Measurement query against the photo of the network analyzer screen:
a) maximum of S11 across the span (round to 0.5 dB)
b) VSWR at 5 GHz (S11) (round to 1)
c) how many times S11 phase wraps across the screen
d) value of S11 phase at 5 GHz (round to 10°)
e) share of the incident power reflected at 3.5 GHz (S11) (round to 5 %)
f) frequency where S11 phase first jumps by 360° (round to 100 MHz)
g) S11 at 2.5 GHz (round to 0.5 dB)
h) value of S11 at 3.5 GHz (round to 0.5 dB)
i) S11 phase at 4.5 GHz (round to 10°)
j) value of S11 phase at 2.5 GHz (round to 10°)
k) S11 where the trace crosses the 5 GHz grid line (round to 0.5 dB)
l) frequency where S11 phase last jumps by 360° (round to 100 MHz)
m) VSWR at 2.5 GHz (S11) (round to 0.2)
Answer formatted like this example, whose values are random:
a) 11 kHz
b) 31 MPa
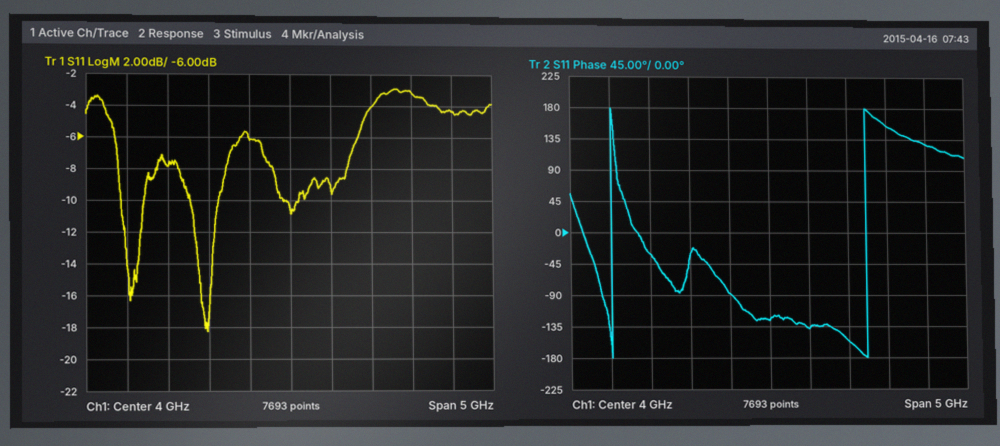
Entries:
a) -3.0 dB
b) 4
c) 2
d) -160°
e) 25 %
f) 2.0 GHz
g) -8.0 dB
h) -6.0 dB
i) -140°
j) -30°
k) -4.0 dB
l) 5.2 GHz
m) 2.4
